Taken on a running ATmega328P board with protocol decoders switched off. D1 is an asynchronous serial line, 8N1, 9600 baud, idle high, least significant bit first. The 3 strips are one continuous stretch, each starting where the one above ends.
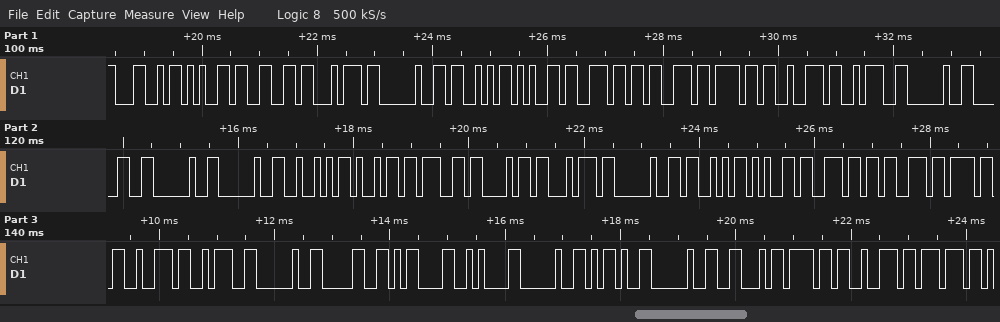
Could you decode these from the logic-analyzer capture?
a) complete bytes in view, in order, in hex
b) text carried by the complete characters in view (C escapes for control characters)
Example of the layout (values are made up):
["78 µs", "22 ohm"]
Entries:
["4C 65 66 74 20 53 65 6E 73 6F 72 3A 20 30 20 20 52 69 67 68 74 20 53 65 6E 73 6F 72 3A 20 30 0D 0A 20 2D 20 46 6F 72 77", "\"Left Sensor: 0  Right Sensor: 0\\r\\n - Forw\""]
